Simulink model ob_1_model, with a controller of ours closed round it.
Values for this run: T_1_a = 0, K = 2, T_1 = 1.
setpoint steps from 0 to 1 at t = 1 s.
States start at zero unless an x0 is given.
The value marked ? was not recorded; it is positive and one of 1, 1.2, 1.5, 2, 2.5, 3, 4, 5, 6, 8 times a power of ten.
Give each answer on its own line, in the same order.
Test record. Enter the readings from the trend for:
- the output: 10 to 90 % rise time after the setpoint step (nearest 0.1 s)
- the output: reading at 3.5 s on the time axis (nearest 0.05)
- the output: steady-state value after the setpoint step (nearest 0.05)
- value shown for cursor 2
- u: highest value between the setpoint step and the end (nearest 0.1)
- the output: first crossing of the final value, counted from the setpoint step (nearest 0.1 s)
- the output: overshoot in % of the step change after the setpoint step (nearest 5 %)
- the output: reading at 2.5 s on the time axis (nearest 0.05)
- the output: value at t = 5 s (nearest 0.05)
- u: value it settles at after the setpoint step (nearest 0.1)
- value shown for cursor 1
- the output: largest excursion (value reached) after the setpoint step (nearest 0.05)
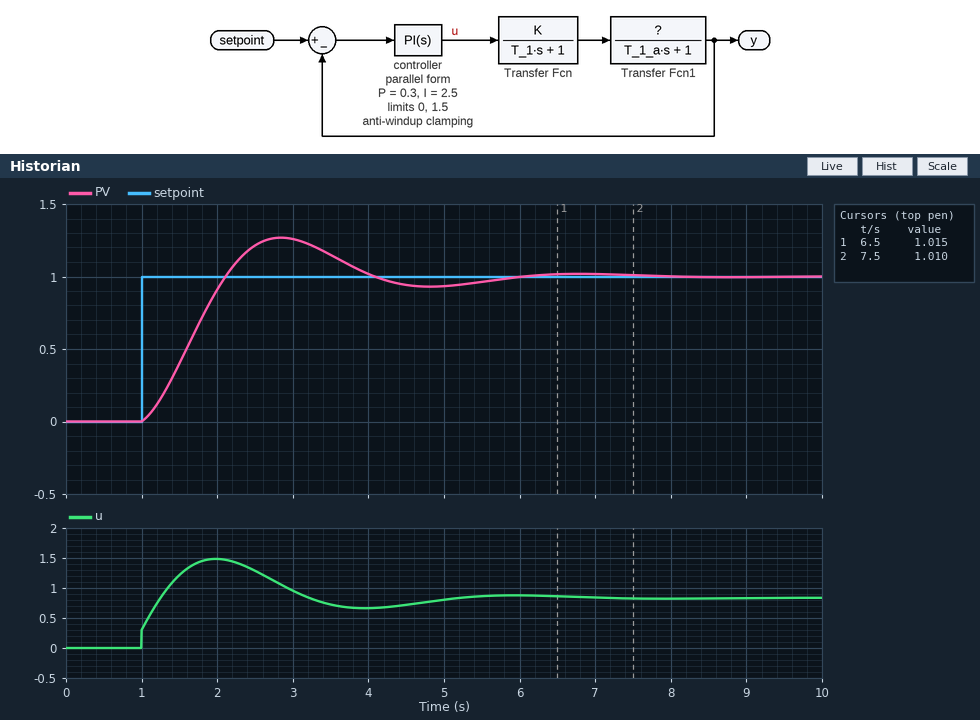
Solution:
0.8 s
1.15
1.00
1.010
1.5
1.1 s
25 %
1.20
0.95
0.8
1.015
1.25
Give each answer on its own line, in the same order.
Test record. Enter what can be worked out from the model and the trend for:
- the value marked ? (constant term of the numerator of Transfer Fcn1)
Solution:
0.6
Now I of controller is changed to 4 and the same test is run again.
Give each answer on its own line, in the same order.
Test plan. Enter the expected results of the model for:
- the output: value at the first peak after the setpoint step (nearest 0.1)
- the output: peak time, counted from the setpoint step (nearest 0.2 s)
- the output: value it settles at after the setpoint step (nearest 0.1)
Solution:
1.2
1.6 s
1.0
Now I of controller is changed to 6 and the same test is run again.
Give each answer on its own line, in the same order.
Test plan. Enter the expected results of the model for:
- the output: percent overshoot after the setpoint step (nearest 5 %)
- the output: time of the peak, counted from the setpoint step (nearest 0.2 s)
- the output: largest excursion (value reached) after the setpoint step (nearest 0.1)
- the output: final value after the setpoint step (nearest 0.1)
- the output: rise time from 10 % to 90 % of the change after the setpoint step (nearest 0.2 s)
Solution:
20 %
1.4 s
1.2
1.0
0.6 s
